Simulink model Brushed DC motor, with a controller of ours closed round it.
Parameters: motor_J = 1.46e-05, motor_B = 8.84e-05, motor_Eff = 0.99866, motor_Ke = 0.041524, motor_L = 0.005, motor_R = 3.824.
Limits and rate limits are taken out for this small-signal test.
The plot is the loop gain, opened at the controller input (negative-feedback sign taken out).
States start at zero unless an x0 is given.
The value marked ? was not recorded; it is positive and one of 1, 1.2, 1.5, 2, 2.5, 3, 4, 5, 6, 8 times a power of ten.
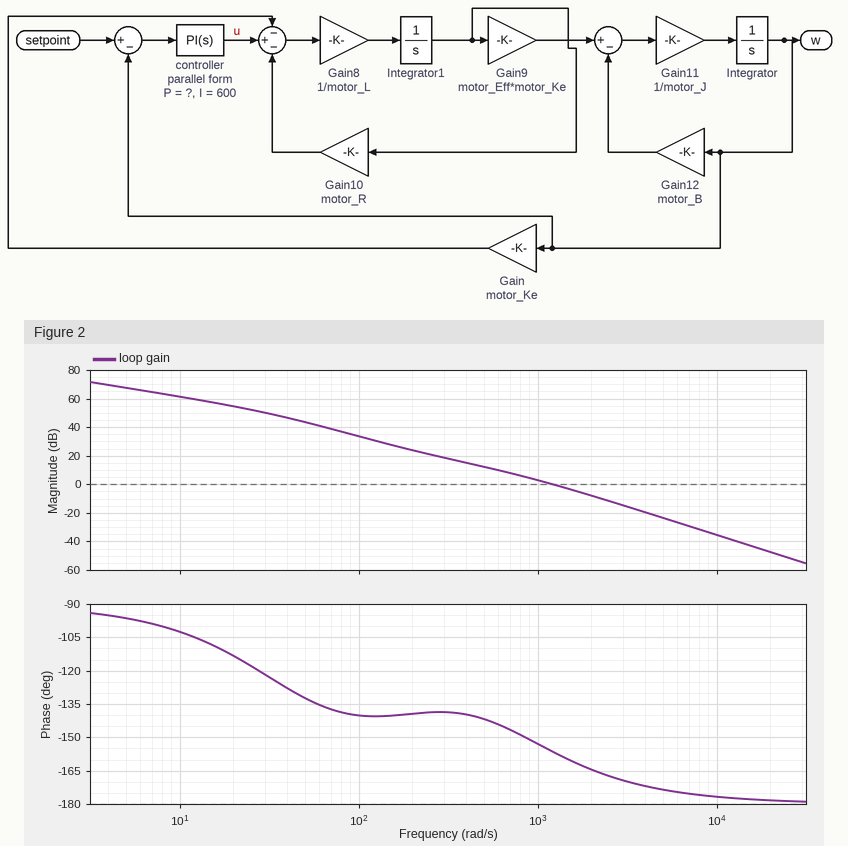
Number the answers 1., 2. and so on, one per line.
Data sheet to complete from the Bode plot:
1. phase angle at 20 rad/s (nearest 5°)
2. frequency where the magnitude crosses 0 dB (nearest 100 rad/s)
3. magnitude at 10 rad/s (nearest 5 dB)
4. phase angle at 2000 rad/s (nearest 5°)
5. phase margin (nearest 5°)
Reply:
1. -115°
2. 1200 rad/s
3. 60 dB
4. -165°
5. 25°
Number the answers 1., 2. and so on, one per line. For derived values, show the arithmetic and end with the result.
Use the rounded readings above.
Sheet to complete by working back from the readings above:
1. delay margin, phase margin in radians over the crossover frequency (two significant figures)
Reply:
1. 25 × π / 180 / 1200 = 0.00036 s
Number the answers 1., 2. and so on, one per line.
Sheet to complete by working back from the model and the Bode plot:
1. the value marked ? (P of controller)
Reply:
1. 3
